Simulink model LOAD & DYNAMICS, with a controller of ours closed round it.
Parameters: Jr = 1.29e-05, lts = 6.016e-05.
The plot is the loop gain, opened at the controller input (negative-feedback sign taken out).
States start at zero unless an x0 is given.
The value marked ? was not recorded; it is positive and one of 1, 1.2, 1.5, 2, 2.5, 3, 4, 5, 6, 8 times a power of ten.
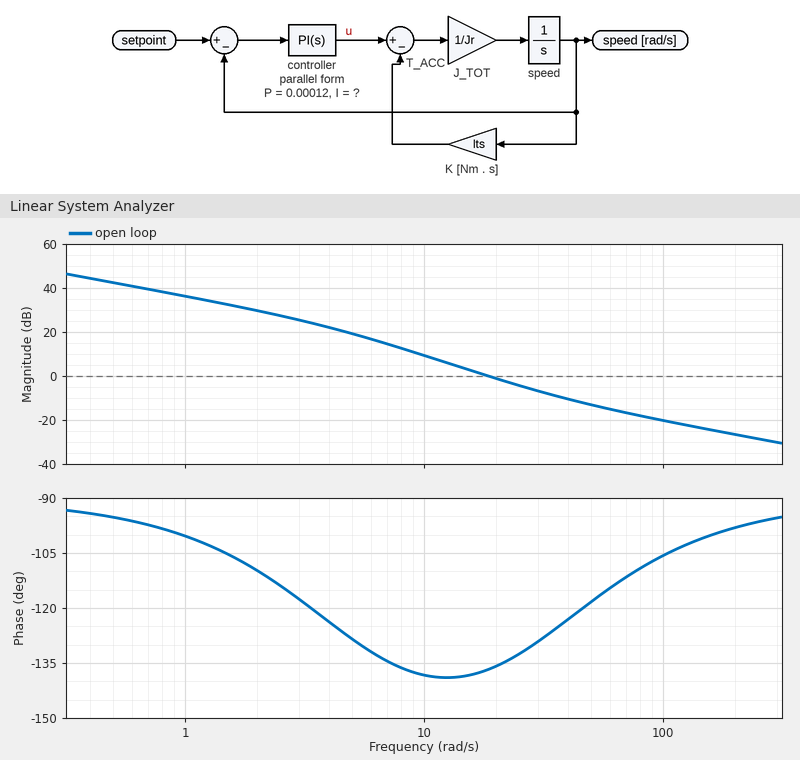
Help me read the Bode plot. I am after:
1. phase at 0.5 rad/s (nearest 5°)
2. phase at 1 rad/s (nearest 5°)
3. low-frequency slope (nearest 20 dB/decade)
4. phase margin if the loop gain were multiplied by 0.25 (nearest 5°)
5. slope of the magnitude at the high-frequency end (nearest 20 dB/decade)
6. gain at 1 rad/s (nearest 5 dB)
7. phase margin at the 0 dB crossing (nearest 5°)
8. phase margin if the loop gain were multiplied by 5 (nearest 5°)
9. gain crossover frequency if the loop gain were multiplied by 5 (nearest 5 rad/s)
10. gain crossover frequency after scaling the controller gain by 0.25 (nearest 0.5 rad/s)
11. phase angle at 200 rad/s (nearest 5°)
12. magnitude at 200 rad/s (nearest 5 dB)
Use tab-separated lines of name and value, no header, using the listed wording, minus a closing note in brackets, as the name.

phase at 0.5 rad/s	-95°
phase at 1 rad/s	-100°
low-frequency slope	-20 dB/decade
phase margin if the loop gain were multiplied by 0.25	45°
slope of the magnitude at the high-frequency end	-20 dB/decade
gain at 1 rad/s	35 dB
phase margin at the 0 dB crossing	45°
phase margin if the loop gain were multiplied by 5	65°
gain crossover frequency if the loop gain were multiplied by 5	55 rad/s
gain crossover frequency after scaling the controller gain by 0.25	8.5 rad/s
phase angle at 200 rad/s	-100°
magnitude at 200 rad/s	-25 dB
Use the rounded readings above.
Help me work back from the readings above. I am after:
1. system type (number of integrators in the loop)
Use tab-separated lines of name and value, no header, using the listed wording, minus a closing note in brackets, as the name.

system type	1
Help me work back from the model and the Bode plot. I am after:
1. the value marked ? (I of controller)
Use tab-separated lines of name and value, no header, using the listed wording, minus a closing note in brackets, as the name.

the value marked ?	0.004
